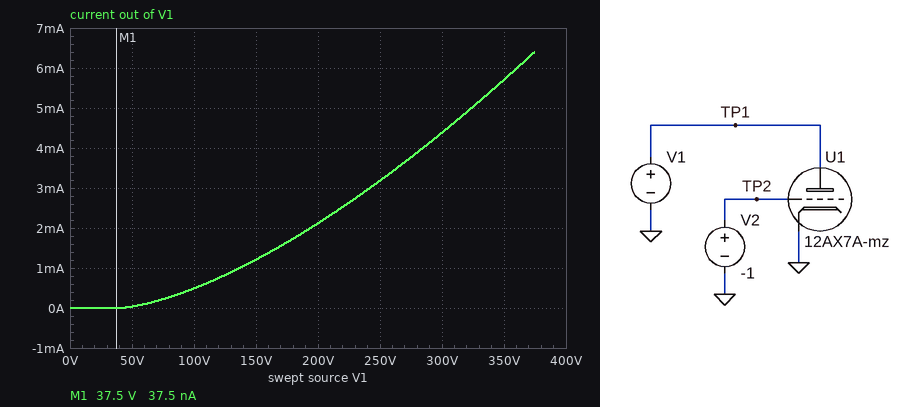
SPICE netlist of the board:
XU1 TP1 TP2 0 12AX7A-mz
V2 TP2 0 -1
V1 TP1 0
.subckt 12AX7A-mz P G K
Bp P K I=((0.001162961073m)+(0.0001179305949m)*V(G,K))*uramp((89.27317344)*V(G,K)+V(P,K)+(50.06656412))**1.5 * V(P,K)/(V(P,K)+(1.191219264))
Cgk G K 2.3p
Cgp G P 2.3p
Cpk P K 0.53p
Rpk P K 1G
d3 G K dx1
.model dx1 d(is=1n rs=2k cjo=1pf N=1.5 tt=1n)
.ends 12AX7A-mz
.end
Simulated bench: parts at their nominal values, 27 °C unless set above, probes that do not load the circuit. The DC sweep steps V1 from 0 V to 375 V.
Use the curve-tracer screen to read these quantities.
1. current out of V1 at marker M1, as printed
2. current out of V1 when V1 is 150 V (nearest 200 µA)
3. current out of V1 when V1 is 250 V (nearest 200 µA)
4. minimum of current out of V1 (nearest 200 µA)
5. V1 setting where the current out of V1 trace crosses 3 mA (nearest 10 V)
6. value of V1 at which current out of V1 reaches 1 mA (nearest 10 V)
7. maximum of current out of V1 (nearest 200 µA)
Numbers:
37.5 nA
1.2 mA
3.2 mA
0 A
240 V
140 V
6.4 mA
